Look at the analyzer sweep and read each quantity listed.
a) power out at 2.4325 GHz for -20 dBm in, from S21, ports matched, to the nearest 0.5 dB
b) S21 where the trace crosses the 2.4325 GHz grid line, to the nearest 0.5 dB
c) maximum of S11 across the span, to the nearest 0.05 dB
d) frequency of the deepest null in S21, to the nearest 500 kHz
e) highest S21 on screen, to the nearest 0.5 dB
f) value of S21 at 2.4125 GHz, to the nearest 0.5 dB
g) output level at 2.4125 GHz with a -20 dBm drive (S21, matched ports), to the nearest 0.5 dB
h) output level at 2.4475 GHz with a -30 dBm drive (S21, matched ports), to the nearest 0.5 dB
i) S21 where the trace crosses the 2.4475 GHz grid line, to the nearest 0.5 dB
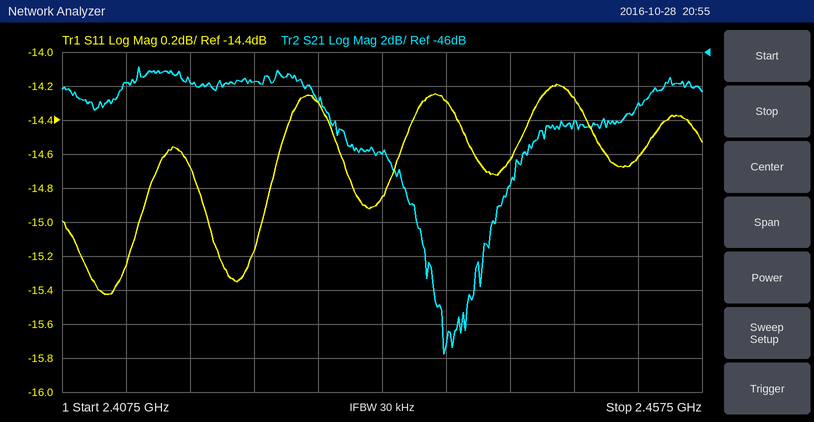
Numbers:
-72.0 dBm
-52.0 dB
-14.20 dB
2.4375 GHz
-47.0 dB
-48.0 dB
-68.0 dBm
-80.0 dBm
-50.0 dB
